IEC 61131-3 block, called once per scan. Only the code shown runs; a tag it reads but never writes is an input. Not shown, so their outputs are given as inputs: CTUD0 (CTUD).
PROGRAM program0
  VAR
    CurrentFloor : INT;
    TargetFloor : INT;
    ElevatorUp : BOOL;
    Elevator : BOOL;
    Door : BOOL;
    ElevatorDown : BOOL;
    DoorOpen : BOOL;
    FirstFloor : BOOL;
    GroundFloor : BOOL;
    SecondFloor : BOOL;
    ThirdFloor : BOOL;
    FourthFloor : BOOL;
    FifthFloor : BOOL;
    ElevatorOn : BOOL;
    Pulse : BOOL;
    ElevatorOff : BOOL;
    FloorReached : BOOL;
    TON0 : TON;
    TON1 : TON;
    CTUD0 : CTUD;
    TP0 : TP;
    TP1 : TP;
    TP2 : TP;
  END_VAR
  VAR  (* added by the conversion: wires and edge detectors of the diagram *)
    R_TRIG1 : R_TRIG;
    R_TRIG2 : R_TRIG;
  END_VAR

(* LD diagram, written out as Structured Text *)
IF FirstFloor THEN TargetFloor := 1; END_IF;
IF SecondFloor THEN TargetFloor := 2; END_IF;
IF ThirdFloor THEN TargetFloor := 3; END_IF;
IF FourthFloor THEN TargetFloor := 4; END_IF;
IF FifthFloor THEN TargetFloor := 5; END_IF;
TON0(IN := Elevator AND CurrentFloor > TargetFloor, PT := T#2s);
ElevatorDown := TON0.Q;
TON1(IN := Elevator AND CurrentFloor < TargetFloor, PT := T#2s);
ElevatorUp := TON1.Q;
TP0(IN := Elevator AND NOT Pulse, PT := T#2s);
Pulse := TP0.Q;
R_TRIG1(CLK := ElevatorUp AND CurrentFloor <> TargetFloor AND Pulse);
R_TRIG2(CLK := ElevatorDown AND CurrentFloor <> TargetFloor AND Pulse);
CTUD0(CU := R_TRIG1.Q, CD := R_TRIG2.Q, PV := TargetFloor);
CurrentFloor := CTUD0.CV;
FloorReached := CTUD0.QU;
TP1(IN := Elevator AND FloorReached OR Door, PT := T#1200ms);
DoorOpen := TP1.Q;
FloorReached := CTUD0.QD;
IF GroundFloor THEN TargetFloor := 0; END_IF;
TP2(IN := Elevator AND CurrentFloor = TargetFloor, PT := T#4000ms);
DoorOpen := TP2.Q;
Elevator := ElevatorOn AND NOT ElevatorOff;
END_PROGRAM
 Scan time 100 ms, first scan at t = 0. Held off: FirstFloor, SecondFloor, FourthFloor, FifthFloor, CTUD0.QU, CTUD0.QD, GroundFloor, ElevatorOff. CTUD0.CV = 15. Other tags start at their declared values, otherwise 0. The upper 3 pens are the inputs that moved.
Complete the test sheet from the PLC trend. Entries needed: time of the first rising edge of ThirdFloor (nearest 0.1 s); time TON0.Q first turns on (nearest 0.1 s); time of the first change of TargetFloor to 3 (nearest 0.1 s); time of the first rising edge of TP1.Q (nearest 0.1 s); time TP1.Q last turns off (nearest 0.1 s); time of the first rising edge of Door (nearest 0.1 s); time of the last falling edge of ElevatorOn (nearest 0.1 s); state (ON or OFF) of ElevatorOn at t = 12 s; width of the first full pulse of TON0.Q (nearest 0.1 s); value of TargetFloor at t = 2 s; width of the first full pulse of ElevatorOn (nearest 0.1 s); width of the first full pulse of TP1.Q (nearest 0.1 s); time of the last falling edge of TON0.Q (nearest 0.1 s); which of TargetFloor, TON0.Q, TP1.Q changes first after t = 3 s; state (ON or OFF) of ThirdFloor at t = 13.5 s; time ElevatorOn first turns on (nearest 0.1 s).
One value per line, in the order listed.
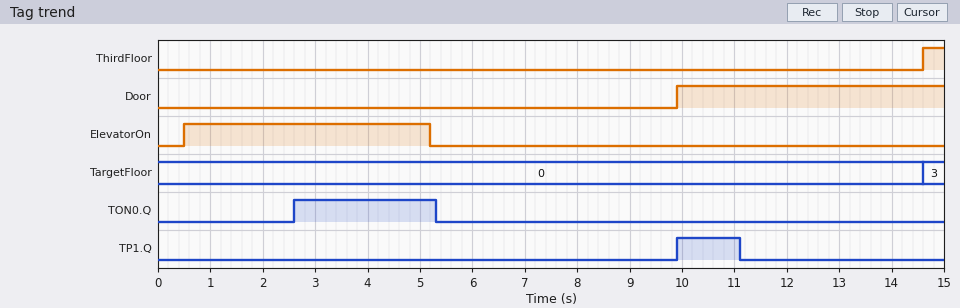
14.6 s
2.6 s
14.6 s
9.9 s
11.1 s
9.9 s
5.2 s
OFF
2.7 s
0
4.7 s
1.2 s
5.3 s
TON0.Q
OFF
0.5 s
